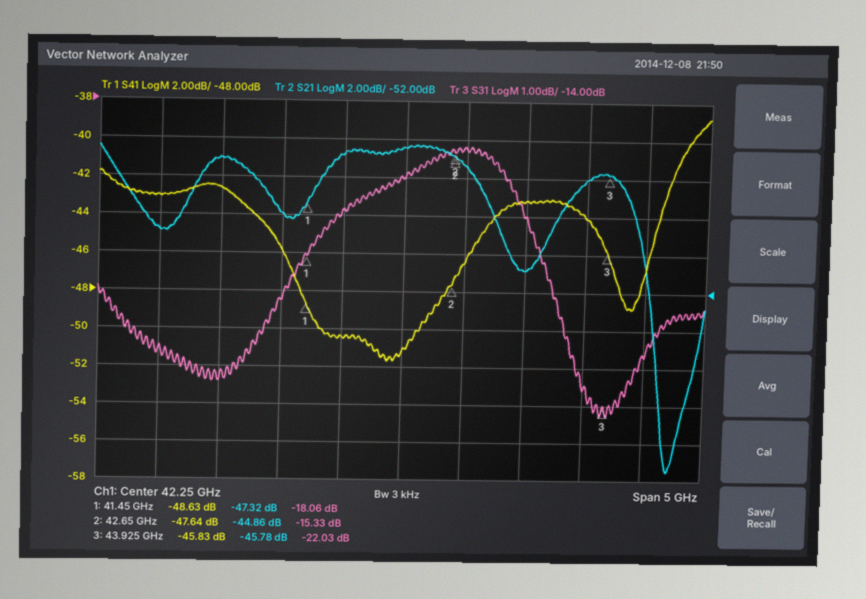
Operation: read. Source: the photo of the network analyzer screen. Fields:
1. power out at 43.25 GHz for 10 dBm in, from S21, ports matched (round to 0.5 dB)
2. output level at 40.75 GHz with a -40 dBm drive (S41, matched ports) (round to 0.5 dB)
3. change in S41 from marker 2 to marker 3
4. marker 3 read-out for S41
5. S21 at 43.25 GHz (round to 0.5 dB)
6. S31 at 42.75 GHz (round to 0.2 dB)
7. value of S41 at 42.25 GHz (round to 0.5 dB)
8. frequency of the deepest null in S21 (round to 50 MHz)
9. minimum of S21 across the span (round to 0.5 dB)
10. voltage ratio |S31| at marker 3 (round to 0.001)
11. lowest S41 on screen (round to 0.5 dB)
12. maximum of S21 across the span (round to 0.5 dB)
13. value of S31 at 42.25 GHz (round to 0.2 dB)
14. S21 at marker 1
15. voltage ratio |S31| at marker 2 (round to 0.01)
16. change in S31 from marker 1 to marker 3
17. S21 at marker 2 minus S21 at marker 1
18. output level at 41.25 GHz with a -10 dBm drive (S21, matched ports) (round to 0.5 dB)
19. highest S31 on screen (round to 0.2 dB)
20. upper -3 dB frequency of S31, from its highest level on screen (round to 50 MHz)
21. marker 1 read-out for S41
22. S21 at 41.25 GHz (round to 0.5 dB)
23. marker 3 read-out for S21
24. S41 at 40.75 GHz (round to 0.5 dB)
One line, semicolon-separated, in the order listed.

-41.0 dBm; -82.5 dBm; 1.81 dB; -45.83 dB; -51.0 dB; -15.2 dB; -51.0 dB; 44.45 GHz; -61.5 dB; 0.079; -51.5 dB; -44.5 dB; -16.0 dB; -47.32 dB; 0.17; -3.97 dB; 2.46 dB; -58.0 dBm; -15.2 dB; 43.40 GHz; -48.63 dB; -48.0 dB; -45.78 dB; -42.5 dB
